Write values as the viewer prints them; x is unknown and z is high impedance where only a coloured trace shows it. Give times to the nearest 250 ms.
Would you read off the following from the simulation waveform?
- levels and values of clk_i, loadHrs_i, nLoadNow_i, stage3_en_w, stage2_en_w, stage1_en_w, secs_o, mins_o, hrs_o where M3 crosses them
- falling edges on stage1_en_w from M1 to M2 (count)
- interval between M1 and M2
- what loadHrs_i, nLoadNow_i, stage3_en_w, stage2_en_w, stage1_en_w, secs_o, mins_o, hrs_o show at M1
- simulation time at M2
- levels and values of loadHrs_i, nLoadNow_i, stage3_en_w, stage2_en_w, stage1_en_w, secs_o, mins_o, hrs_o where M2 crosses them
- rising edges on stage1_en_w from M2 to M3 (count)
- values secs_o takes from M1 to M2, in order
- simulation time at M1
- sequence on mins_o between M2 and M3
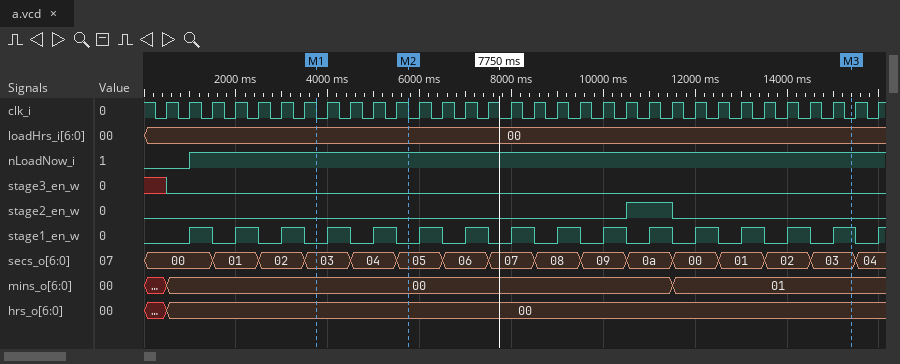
clk_i=0, loadHrs_i=00, nLoadNow_i=1, stage3_en_w=0, stage2_en_w=0, stage1_en_w=1, secs_o=03, mins_o=01, hrs_o=00
2
2000 ms
loadHrs_i=00, nLoadNow_i=1, stage3_en_w=0, stage2_en_w=0, stage1_en_w=0, secs_o=03, mins_o=00, hrs_o=00
5750 ms
loadHrs_i=00, nLoadNow_i=1, stage3_en_w=0, stage2_en_w=0, stage1_en_w=0, secs_o=05, mins_o=00, hrs_o=00
10
03, 04, 05
3750 ms
00, 01
